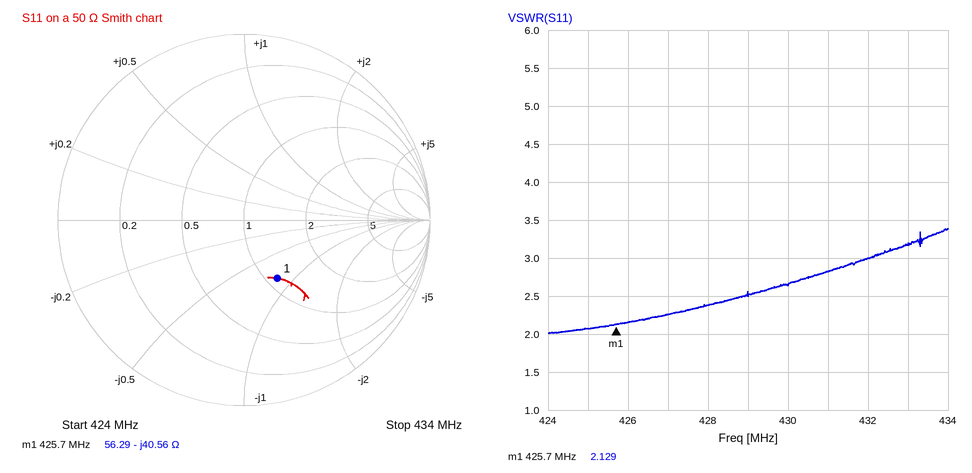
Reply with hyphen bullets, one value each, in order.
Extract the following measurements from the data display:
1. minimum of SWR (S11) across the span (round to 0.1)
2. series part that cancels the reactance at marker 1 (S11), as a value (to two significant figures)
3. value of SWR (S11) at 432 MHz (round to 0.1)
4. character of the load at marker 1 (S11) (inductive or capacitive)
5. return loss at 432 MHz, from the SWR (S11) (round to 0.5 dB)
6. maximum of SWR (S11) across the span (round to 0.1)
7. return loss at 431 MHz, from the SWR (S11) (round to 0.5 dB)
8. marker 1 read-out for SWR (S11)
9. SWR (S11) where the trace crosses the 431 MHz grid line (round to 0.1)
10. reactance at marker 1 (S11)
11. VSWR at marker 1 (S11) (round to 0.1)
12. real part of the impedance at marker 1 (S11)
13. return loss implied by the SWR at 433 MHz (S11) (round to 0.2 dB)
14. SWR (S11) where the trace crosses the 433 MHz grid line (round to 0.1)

- 2.0
- 15 nH
- 3.0
- capacitive
- 6.0 dB
- 3.4
- 6.5 dB
- 2.129
- 2.8
- -40.56 Ω
- 2.1
- 56.29 Ω
- 5.6 dB
- 3.2
